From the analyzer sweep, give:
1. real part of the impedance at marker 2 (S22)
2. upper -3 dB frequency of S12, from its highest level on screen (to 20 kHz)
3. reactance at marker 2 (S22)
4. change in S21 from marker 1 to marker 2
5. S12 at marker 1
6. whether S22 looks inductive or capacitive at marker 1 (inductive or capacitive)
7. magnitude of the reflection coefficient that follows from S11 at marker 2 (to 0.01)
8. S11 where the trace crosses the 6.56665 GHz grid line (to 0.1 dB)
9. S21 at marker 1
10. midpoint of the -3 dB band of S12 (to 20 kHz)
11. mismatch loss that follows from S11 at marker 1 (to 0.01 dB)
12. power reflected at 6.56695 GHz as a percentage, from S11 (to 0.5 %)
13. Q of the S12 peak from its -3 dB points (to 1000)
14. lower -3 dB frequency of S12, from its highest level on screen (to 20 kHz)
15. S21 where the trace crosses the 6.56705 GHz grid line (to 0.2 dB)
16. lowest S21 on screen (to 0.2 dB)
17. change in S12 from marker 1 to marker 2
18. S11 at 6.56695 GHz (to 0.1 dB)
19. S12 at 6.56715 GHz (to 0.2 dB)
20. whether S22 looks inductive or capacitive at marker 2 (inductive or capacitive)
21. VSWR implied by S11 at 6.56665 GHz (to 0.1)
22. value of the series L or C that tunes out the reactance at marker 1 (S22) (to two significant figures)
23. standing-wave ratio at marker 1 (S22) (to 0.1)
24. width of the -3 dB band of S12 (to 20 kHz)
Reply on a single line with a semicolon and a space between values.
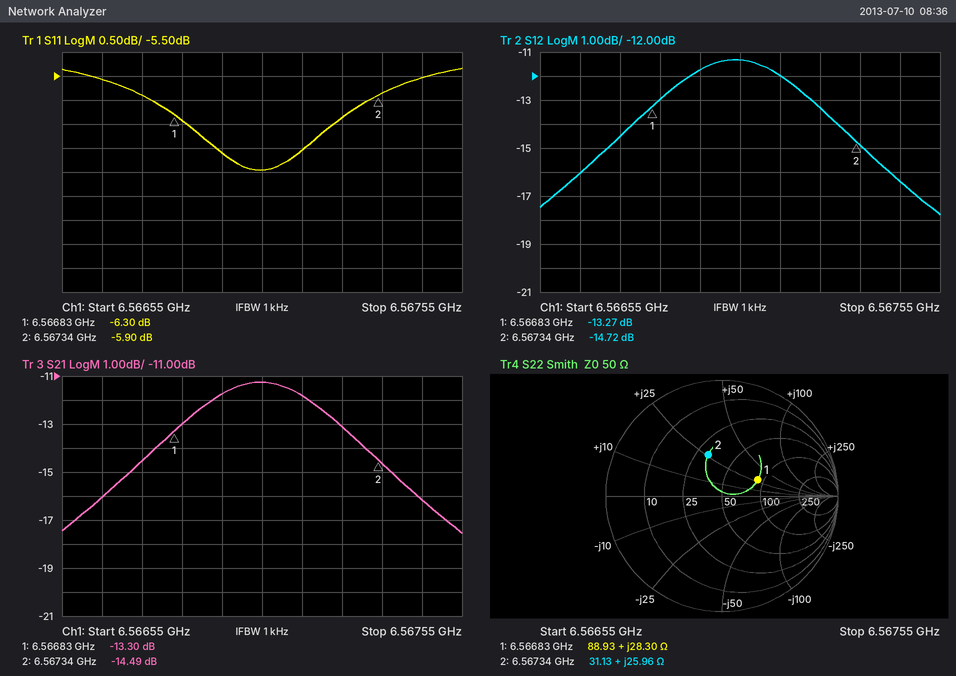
31.13 Ω; 6.56732 GHz; +25.96 Ω; -1.19 dB; -13.27 dB; inductive; 0.51; -5.6 dB; -13.30 dB; 6.56704 GHz; 1.16 dB; 19.5 %; 12000; 6.56676 GHz; -11.2 dB; -17.6 dB; -1.45 dB; -7.1 dB; -12.0 dB; inductive; 3.2; 860 fF; 2.0; 560 kHz
